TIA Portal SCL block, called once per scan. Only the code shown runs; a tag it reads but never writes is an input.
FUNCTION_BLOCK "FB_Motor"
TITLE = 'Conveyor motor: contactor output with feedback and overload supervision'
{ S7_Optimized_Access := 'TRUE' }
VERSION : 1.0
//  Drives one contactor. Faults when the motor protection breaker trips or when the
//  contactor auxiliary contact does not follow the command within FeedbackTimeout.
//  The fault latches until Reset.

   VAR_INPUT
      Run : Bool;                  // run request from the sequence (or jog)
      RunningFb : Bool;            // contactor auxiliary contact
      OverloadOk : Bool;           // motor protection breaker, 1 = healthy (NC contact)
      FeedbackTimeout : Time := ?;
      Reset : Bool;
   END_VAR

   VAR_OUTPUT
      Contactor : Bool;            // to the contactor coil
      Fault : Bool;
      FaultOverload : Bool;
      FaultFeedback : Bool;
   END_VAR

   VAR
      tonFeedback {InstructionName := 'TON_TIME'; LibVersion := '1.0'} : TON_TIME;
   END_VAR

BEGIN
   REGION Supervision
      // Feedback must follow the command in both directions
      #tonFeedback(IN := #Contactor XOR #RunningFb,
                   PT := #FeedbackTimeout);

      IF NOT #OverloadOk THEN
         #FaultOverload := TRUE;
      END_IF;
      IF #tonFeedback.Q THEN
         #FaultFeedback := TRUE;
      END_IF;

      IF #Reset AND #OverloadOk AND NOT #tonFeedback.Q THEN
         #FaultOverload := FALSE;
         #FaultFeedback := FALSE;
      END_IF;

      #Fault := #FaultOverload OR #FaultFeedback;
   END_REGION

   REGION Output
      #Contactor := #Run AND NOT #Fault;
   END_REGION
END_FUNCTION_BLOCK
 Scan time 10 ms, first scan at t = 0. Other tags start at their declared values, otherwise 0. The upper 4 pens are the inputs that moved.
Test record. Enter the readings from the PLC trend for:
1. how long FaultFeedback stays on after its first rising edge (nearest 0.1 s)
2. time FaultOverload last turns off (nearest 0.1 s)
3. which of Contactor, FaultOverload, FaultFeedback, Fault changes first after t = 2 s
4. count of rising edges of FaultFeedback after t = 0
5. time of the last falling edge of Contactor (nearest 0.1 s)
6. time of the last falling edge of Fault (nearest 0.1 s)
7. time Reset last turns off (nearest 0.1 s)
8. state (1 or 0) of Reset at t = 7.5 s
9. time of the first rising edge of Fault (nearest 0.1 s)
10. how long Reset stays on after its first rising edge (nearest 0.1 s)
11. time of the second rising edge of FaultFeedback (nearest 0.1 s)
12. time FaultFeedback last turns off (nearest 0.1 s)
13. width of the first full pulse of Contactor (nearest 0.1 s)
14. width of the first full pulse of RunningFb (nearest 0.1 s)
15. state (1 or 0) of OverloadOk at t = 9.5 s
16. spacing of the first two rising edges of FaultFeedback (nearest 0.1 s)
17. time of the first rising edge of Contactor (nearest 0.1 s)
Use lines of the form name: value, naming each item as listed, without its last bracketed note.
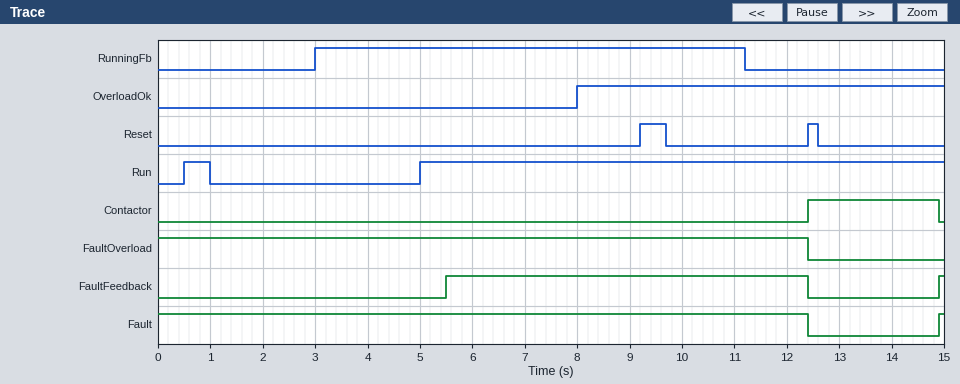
how long FaultFeedback stays on after its first rising edge: 6.9 s
time FaultOverload last turns off: 12.4 s
which of Contactor, FaultOverload, FaultFeedback, Fault changes first after t = 2 s: FaultFeedback
count of rising edges of FaultFeedback after t = 0: 2
time of the last falling edge of Contactor: 14.9 s
time of the last falling edge of Fault: 12.4 s
time Reset last turns off: 12.6 s
state (1 or 0) of Reset at t = 7.5 s: 0
time of the first rising edge of Fault: 14.9 s
how long Reset stays on after its first rising edge: 0.5 s
time of the second rising edge of FaultFeedback: 14.9 s
time FaultFeedback last turns off: 12.4 s
width of the first full pulse of Contactor: 2.5 s
width of the first full pulse of RunningFb: 8.2 s
state (1 or 0) of OverloadOk at t = 9.5 s: 1
spacing of the first two rising edges of FaultFeedback: 9.4 s
time of the first rising edge of Contactor: 12.4 s
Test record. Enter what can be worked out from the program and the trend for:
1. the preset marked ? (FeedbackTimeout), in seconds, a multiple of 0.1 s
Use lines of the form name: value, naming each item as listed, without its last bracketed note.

the preset marked ? (FeedbackTimeout), in seconds, a multiple of 0.1 s: 2.5 s
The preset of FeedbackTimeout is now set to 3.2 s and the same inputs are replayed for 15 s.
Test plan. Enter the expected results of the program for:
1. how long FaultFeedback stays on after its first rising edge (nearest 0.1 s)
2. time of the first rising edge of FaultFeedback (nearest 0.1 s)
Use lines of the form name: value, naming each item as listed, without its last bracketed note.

how long FaultFeedback stays on after its first rising edge: 6.2 s
time of the first rising edge of FaultFeedback: 6.2 s
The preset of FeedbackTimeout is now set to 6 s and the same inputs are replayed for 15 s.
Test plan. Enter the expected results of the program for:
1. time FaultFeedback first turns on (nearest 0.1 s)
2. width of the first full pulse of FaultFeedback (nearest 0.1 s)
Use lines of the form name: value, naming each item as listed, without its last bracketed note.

time FaultFeedback first turns on: 9.0 s
width of the first full pulse of FaultFeedback: 3.4 s
